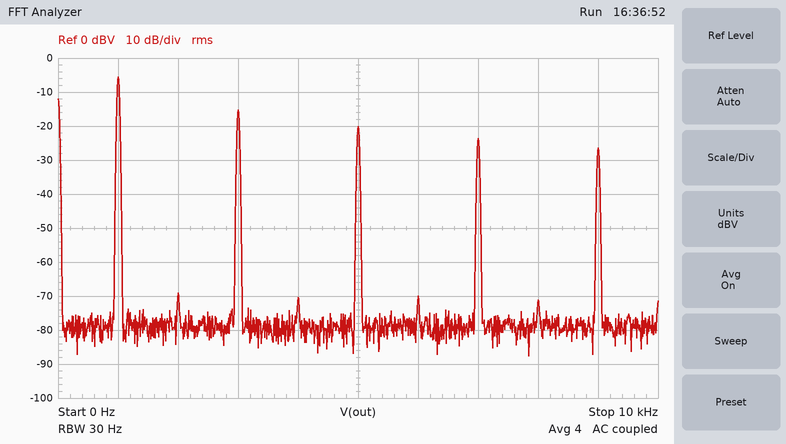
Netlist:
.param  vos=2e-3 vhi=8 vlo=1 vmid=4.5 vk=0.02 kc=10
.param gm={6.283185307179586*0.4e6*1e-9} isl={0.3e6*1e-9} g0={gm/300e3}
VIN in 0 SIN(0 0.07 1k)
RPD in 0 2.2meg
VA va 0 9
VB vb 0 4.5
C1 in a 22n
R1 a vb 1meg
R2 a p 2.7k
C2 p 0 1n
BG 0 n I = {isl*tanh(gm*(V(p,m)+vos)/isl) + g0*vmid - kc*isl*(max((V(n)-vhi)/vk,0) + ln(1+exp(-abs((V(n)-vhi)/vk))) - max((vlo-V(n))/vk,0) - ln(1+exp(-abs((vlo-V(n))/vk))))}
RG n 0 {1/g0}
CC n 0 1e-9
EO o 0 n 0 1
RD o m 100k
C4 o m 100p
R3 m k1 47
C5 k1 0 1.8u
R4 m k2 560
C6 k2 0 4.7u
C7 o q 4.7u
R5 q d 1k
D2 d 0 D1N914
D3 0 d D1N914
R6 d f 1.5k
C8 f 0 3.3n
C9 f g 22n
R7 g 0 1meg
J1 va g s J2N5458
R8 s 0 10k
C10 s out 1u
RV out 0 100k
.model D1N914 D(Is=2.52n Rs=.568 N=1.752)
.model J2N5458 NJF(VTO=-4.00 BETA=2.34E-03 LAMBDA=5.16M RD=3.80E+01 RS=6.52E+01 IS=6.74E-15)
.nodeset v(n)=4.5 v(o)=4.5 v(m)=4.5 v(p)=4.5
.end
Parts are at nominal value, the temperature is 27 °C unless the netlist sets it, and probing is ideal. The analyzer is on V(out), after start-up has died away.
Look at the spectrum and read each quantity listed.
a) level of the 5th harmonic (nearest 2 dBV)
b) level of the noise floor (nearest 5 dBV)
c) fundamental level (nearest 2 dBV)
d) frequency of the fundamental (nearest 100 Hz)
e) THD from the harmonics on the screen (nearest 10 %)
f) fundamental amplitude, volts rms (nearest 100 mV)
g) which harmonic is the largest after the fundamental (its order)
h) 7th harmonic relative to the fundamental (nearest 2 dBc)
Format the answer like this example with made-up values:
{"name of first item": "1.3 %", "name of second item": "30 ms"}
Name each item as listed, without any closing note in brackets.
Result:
{"level of the 5th harmonic": "-20 dBV", "level of the noise floor": "-80 dBV", "fundamental level": "-6 dBV", "frequency of the fundamental": "1.0 kHz", "THD from the harmonics on the screen": "40 %", "fundamental amplitude, volts rms": "500 mV", "which harmonic is the largest after the fundamental": "3", "7th harmonic relative to the fundamental": "-18 dBc"}
